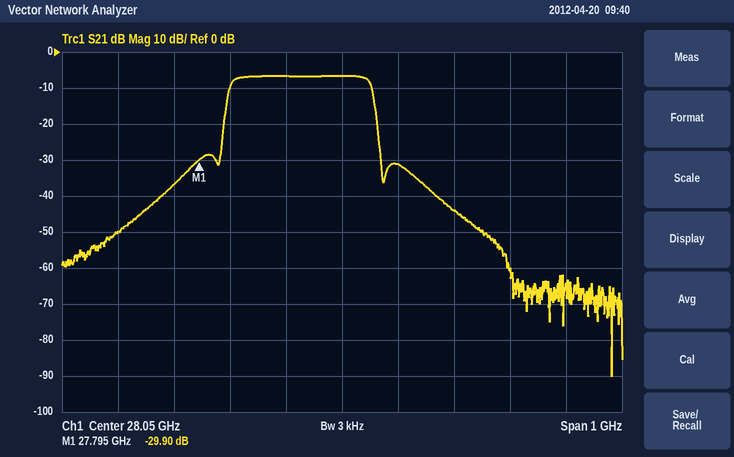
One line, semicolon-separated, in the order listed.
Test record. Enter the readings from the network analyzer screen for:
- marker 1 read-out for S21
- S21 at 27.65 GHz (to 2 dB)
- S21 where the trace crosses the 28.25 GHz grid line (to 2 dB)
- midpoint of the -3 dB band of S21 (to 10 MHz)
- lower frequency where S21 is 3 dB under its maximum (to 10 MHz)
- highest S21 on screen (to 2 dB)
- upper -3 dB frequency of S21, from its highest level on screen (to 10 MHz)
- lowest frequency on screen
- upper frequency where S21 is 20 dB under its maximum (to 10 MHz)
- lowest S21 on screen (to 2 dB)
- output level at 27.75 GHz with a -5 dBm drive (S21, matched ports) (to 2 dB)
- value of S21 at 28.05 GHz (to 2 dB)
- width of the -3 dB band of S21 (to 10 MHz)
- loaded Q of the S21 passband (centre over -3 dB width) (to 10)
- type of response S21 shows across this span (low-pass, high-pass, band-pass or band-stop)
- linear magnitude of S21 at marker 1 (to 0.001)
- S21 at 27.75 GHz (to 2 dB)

-29.90 dB; -50 dB; -44 dB; 27.98 GHz; 27.85 GHz; -6 dB; 28.10 GHz; 27.55 GHz; 28.12 GHz; -90 dB; -42 dBm; -6 dB; 250 MHz; 110; band-pass; 0.032; -36 dB
